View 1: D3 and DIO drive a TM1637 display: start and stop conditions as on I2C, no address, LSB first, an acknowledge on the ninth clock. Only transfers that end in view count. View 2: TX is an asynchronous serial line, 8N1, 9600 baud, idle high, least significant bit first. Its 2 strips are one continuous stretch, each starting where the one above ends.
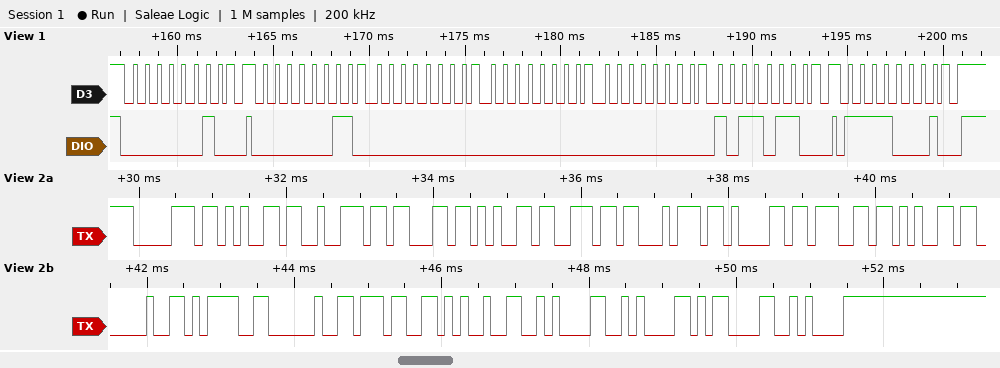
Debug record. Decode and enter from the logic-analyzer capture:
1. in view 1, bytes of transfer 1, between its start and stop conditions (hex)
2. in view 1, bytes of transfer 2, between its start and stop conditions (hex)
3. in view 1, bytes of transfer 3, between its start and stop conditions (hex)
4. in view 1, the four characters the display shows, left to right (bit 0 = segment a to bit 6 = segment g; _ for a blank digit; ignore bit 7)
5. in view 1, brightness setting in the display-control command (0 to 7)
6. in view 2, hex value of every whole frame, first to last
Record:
40
C0 00 00 00 6D
8F
___5
7
0x70 0x65 0x72 0x63 0x65 0x6E 0x74 0x61 0x67 0x65 0x20 0x3D 0x20 0x37 0x25 0x0A 0x0A 0x0D 0x0A
